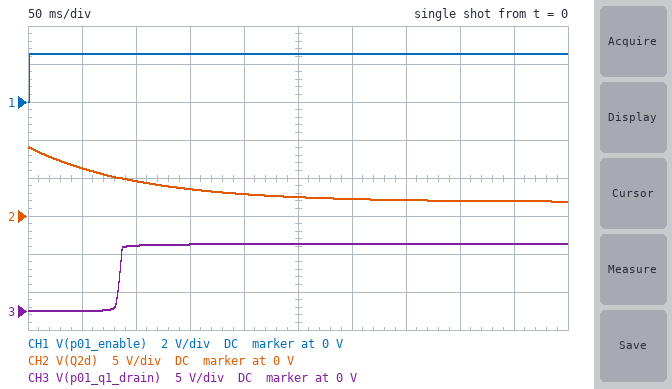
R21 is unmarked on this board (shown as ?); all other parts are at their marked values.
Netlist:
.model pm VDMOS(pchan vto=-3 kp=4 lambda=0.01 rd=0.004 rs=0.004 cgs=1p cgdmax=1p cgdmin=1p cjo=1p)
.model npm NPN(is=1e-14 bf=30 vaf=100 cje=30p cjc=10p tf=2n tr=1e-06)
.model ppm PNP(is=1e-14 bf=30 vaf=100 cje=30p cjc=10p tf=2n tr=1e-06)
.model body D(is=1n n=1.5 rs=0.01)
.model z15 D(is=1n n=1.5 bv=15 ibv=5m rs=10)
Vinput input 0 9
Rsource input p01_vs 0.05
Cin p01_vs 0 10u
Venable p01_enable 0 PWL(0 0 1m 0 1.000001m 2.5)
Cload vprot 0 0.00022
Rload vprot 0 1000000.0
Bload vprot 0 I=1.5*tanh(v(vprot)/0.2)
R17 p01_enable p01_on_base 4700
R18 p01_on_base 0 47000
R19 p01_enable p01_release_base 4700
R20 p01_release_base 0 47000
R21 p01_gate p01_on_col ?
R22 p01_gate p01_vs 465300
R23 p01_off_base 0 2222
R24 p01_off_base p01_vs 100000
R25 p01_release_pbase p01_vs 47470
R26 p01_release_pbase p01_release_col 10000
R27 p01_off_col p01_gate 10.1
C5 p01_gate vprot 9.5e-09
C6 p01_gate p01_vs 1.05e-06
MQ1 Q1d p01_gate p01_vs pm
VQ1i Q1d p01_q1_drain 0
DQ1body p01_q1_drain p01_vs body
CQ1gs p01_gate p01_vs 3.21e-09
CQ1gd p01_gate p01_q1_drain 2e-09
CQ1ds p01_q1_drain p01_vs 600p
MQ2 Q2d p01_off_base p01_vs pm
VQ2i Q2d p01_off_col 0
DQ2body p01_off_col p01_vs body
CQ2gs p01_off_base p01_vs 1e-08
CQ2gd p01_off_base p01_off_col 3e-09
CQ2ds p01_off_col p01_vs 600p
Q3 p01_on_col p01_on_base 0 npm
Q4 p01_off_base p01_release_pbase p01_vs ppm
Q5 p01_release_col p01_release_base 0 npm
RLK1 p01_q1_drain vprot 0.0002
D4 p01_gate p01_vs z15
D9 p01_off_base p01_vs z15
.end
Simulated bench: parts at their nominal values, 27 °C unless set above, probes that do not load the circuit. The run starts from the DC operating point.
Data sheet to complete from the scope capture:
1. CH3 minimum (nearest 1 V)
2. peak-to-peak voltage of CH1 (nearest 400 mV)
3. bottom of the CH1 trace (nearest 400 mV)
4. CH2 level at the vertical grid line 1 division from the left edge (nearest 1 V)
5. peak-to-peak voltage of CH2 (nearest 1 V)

0 V
2.4 V
0 V
6 V
7 V
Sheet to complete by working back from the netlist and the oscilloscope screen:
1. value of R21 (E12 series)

120 kΩ
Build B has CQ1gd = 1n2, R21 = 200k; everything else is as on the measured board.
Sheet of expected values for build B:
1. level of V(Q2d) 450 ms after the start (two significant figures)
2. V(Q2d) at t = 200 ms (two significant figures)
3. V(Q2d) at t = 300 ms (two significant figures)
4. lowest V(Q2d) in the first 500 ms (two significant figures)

3.0 V
4.4 V
3.6 V
2.9 V
